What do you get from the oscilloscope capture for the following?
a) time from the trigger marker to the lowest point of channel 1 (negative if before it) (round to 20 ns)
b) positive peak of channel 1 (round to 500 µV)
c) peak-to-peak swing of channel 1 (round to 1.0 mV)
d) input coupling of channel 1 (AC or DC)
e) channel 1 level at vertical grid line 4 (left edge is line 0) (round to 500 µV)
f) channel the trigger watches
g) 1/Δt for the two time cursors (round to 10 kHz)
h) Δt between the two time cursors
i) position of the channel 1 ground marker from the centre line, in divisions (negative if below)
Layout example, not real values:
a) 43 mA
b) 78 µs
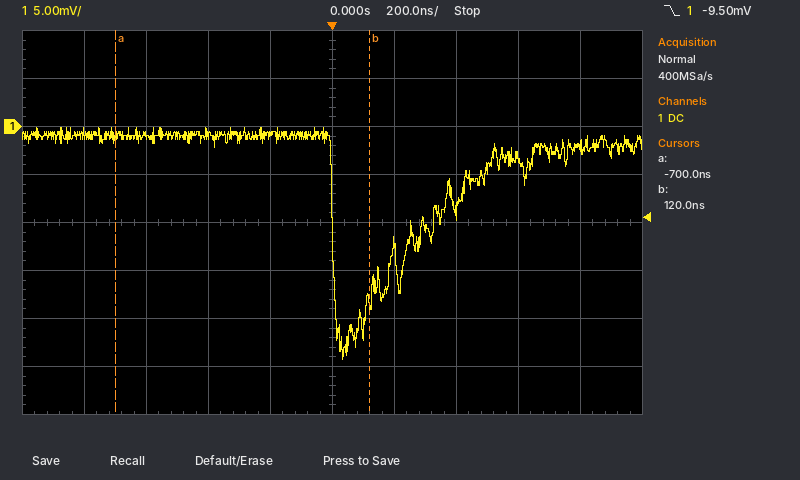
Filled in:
a) +40 ns
b) 0.0 mV
c) 24.0 mV
d) DC
e) -1.0 mV
f) channel 1
g) 1.22 MHz
h) 820 ns
i) +2.0 div
